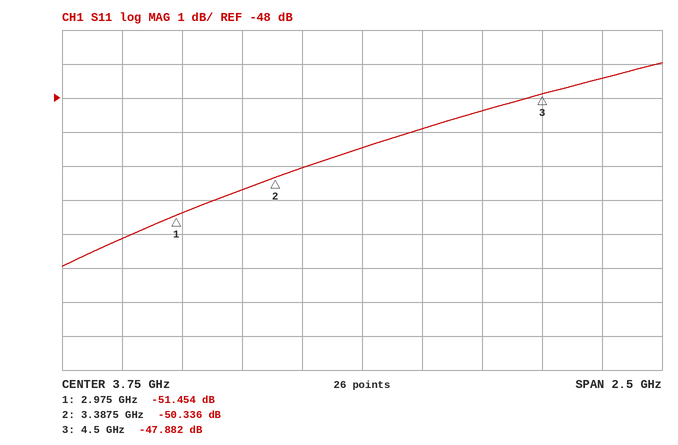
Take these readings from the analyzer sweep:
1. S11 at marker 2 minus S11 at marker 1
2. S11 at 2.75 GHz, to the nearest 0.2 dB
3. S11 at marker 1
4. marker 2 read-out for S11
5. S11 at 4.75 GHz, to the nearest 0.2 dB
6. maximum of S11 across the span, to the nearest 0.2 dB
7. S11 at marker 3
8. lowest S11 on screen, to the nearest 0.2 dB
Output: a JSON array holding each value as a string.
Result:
["1.118 dB", "-52.2 dB", "-51.454 dB", "-50.336 dB", "-47.4 dB", "-47.0 dB", "-47.882 dB", "-53.0 dB"]
